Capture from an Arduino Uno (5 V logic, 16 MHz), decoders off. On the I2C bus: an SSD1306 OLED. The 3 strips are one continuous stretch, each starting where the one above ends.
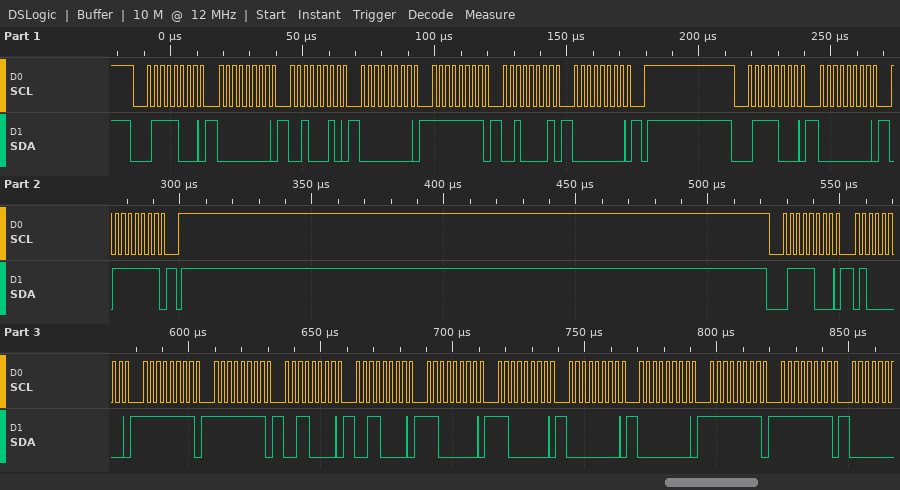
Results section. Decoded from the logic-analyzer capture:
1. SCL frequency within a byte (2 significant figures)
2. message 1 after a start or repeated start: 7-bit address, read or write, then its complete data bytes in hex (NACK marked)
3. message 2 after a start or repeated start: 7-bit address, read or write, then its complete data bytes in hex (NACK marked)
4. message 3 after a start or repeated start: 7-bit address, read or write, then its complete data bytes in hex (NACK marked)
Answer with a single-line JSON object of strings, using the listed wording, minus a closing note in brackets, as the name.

{"SCL frequency within a byte": "400 kHz", "message 1 after a start or repeated start: 7-bit address, read or write, then its complete data bytes in hex": "0x3C write: 00 22 00 FF 21 00", "message 2 after a start or repeated start: 7-bit address, read or write, then its complete data bytes in hex": "0x3C write: 00 7F", "message 3 after a start or repeated start: 7-bit address, read or write, then its complete data bytes in hex": "0x3C write: 40 FF FF 30 30 C0 C0 00 00 FF FF"}
